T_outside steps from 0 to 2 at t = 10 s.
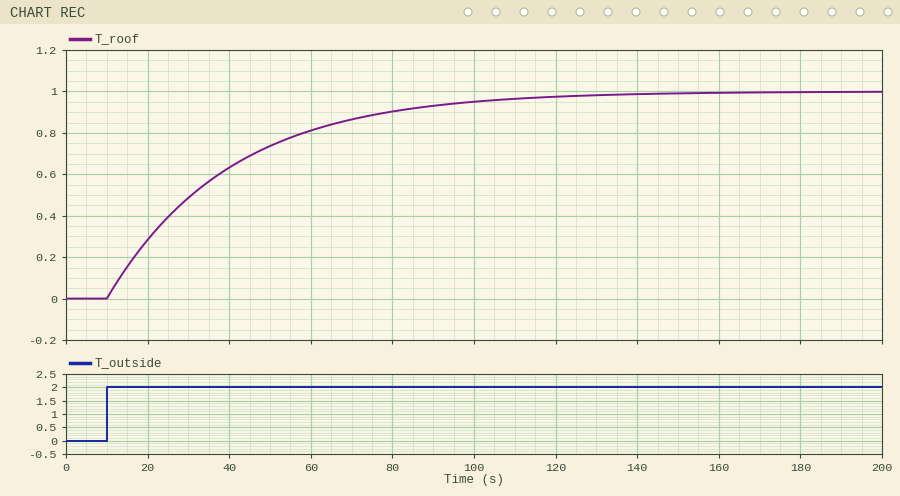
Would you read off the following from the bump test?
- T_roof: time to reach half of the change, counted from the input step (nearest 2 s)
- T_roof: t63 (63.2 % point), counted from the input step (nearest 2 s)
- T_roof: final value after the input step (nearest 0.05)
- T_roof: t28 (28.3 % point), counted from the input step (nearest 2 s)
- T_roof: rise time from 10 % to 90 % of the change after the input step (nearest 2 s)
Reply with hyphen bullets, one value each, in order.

- 20 s
- 30 s
- 1.00
- 10 s
- 66 s
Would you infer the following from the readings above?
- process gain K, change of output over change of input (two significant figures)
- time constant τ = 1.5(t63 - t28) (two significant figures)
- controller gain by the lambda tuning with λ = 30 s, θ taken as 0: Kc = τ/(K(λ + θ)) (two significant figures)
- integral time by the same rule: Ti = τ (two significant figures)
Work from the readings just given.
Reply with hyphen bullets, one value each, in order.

- 0.50
- 30 s
- 2.0
- 30 s
